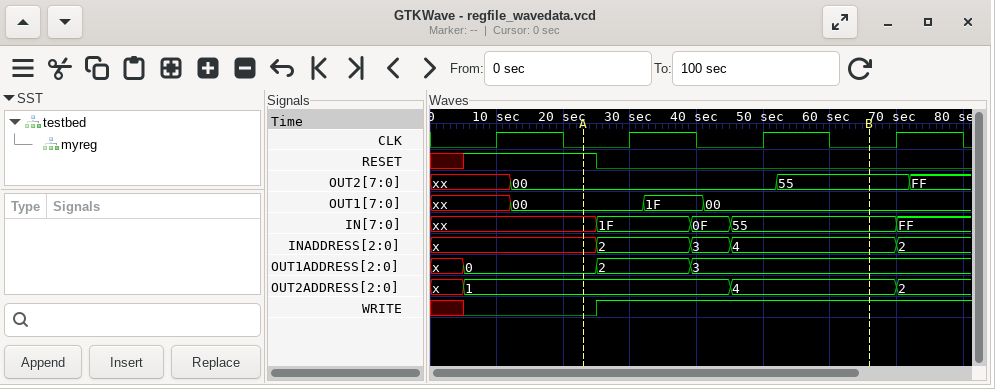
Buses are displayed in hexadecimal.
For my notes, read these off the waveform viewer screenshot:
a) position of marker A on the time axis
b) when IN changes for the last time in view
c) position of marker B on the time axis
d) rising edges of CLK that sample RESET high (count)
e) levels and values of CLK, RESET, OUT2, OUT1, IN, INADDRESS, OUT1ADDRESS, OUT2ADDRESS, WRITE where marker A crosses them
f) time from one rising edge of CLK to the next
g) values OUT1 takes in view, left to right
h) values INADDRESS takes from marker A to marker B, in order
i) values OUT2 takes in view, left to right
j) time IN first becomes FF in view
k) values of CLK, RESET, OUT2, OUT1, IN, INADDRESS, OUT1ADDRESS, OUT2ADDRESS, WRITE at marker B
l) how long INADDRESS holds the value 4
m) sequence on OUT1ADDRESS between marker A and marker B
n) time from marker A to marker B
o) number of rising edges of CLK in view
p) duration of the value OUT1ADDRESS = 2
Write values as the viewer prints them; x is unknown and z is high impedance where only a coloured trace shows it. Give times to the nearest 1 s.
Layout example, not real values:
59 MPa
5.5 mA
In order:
23 s
70 s
66 s
1
CLK=0, RESET=1, OUT2=00, OUT1=00, IN=xx, INADDRESS=x, OUT1ADDRESS=0, OUT2ADDRESS=1, WRITE=0
20 s
xx, 00, 1F, 00
x, 2, 3, 4
xx, 00, 55, FF
70 s
CLK=0, RESET=0, OUT2=55, OUT1=00, IN=55, INADDRESS=4, OUT1ADDRESS=3, OUT2ADDRESS=4, WRITE=1
25 s
0, 2, 3
43 s
4
14 s
